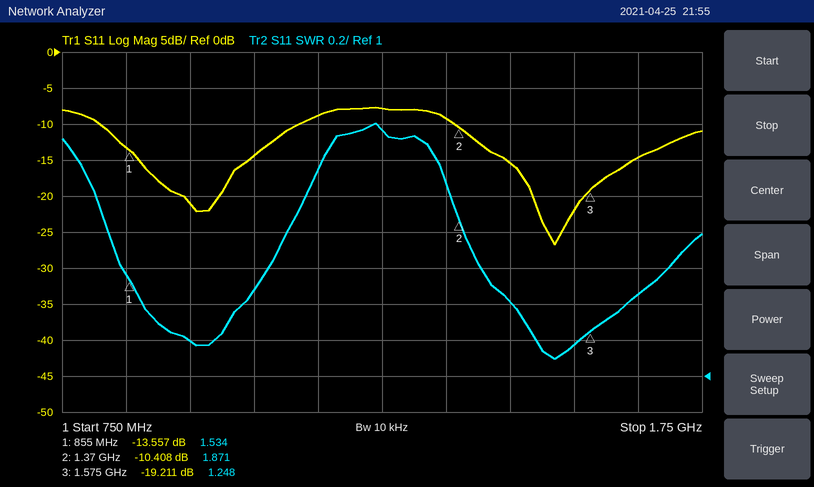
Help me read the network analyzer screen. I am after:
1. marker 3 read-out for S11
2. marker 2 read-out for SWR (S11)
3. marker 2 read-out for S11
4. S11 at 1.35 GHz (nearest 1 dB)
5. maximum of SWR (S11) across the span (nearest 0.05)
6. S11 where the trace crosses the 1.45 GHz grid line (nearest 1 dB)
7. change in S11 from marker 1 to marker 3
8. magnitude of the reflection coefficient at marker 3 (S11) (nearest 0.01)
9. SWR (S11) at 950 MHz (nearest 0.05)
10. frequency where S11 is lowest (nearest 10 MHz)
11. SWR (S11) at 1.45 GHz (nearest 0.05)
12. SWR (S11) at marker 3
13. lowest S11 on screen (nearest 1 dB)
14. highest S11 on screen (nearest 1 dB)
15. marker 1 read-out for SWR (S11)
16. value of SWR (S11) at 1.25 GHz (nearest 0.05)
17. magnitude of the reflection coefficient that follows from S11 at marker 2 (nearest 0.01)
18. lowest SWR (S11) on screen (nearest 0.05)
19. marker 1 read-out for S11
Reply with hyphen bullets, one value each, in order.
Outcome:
- -19.211 dB
- 1.871
- -10.408 dB
- -9 dB
- 2.40
- -15 dB
- -5.654 dB
- 0.11
- 1.20
- 1.52 GHz
- 1.40
- 1.248
- -27 dB
- -8 dB
- 1.534
- 2.35
- 0.30
- 1.10
- -13.557 dB
